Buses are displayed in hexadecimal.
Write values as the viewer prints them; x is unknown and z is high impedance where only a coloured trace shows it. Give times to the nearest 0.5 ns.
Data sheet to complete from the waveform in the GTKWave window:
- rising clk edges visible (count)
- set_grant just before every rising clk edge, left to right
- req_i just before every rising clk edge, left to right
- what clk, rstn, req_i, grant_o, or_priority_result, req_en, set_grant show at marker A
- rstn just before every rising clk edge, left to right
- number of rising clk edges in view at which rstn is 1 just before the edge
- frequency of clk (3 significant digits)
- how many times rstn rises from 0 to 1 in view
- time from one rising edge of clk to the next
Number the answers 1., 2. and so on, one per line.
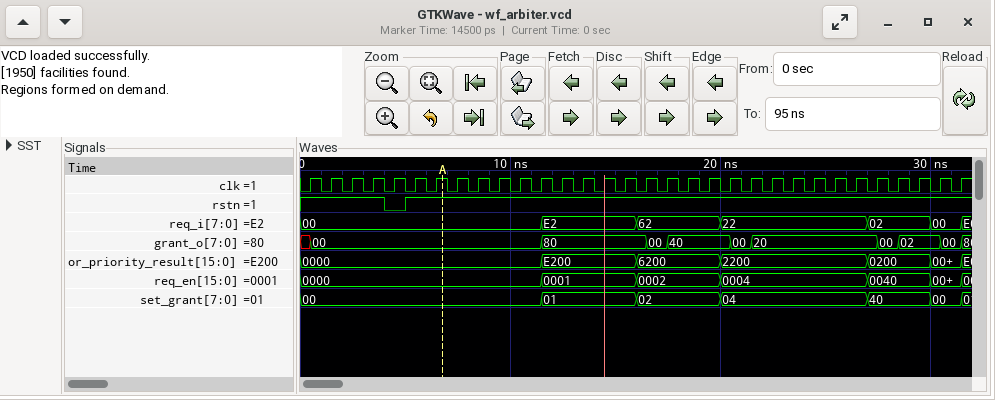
1. 32
2. 00, 00, 00, 00, 00, 00, 00, 00, 00, 00, 00, 00, 01, 01, 01, 01, 02, 02, 02, 02, 04, 04, 04, 04, 04, 04, 04, 40, 40, 40, 00, 00
3. 00, 00, 00, 00, 00, 00, 00, 00, 00, 00, 00, 00, E2, E2, E2, E2, 62, 62, 62, 62, 22, 22, 22, 22, 22, 22, 22, 02, 02, 02, 00, 00
4. clk=1, rstn=1, req_i=00, grant_o=00, or_priority_result=0000, req_en=0000, set_grant=00
5. 1 1 1 1 0 1 1 1 1 1 1 1 1 1 1 1 1 1 1 1 1 1 1 1 1 1 1 1 1 1 1 1
6. 31
7. 1.00 GHz
8. 1
9. 1 ns
